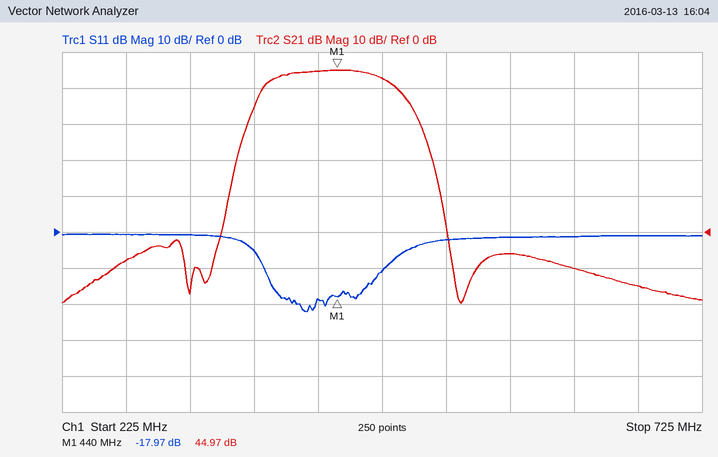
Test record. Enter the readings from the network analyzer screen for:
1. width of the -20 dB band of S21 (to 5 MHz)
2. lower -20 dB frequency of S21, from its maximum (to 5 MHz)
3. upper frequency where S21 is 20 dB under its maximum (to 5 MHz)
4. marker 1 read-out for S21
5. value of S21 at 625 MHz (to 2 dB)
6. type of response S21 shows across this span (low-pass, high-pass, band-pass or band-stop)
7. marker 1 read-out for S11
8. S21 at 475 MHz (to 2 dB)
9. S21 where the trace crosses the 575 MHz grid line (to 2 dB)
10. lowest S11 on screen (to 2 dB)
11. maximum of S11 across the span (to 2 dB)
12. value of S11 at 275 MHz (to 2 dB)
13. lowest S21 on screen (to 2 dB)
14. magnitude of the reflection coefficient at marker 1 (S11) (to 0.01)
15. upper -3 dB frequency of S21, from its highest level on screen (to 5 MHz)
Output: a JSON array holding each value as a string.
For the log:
["145 MHz", "365 MHz", "510 MHz", "44.97 dB", "-10 dB", "band-pass", "-17.97 dB", "42 dB", "-6 dB", "-22 dB", "0 dB", "0 dB", "-20 dB", "0.13", "480 MHz"]
